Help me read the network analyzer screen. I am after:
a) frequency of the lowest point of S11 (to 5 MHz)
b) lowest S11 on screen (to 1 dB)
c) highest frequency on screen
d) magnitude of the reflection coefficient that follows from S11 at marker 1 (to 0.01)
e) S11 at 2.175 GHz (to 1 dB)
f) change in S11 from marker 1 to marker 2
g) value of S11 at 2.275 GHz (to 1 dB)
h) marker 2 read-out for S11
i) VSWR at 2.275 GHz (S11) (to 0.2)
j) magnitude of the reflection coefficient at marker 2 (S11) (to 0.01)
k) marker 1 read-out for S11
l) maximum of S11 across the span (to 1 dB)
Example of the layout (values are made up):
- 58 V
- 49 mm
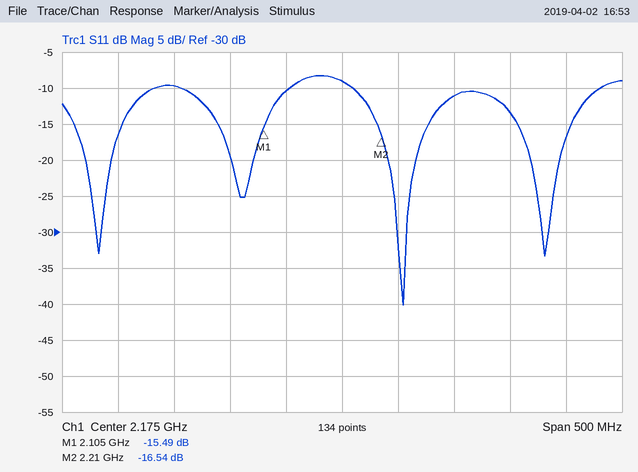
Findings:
- 2.230 GHz
- -40 dB
- 2.425 GHz
- 0.17
- -9 dB
- -1.05 dB
- -11 dB
- -16.54 dB
- 1.8
- 0.15
- -15.49 dB
- -8 dB
